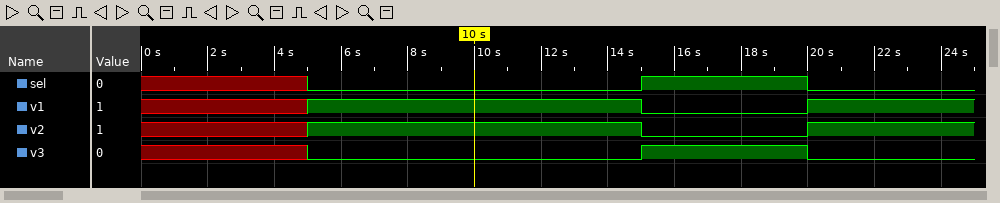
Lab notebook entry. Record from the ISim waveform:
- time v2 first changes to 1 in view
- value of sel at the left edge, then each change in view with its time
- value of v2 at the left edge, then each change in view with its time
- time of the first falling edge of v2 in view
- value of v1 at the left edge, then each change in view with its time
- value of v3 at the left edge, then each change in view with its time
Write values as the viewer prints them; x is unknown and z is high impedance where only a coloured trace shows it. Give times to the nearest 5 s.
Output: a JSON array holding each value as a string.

["5 s", "x, 0 at 5 s, 1 at 15 s, 0 at 20 s", "x, 1 at 5 s, 0 at 15 s, 1 at 20 s", "15 s", "x, 1 at 5 s, 0 at 15 s, 1 at 20 s", "x, 0 at 5 s, 1 at 15 s, 0 at 20 s"]
